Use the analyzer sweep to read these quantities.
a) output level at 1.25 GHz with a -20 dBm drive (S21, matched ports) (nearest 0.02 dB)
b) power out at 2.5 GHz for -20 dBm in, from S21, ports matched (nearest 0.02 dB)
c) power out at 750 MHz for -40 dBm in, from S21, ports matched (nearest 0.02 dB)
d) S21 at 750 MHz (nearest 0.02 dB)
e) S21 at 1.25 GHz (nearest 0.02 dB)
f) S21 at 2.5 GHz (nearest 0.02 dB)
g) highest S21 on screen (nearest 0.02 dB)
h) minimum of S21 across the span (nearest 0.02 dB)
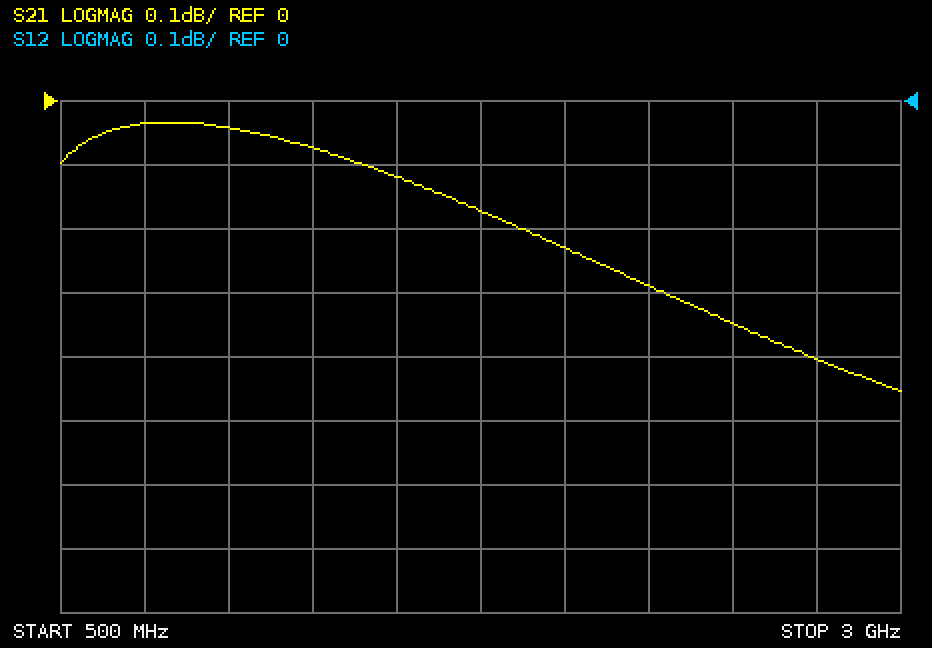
-20.08 dBm
-20.34 dBm
-40.04 dBm
-0.04 dB
-0.08 dB
-0.34 dB
-0.04 dB
-0.46 dB
